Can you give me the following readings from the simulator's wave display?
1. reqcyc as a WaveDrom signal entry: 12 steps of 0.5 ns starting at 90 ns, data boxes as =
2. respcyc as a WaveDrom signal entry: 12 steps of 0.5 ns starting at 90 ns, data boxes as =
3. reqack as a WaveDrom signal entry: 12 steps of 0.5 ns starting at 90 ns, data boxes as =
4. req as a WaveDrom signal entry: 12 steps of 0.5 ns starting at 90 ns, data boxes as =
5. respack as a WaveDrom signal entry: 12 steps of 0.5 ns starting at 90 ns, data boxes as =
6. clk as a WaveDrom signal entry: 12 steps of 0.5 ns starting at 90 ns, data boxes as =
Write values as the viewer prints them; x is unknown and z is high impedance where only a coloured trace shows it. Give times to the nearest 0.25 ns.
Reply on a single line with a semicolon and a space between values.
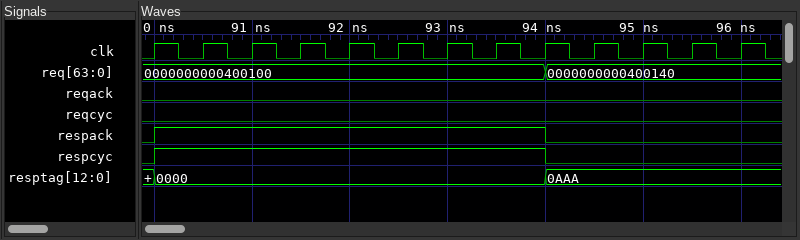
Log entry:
{name: 'reqcyc', wave: '0...........'}; {name: 'respcyc', wave: '1.......0...'}; {name: 'reqack', wave: '0...........'}; {name: 'req', wave: '=.......=...', data: '0000000000400100 0000000000400140'}; {name: 'respack', wave: '1.......0...'}; {name: 'clk', wave: 'p...........'}
